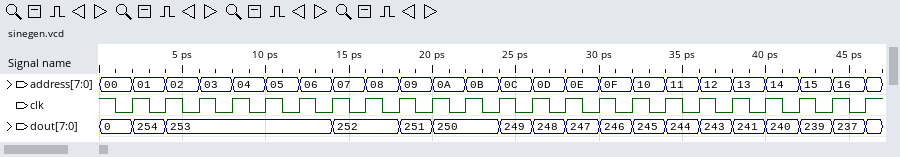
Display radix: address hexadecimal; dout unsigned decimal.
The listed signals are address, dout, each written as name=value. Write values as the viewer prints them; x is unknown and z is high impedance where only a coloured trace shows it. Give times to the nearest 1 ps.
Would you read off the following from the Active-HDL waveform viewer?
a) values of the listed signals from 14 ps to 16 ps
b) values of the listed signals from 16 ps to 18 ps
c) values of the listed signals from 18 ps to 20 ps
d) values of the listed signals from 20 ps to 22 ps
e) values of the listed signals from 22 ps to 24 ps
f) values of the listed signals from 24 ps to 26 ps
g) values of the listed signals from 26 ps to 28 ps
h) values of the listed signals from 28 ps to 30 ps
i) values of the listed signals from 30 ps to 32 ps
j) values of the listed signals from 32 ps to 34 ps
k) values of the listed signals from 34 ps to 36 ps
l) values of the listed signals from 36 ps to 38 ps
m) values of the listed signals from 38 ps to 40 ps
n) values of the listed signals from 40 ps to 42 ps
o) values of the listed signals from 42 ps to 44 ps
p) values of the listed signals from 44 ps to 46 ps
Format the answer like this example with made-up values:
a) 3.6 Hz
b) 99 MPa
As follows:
a) address=07, dout=252
b) address=08, dout=252
c) address=09, dout=251
d) address=0A, dout=250
e) address=0B, dout=250
f) address=0C, dout=249
g) address=0D, dout=248
h) address=0E, dout=247
i) address=0F, dout=246
j) address=10, dout=245
k) address=11, dout=244
l) address=12, dout=243
m) address=13, dout=241
n) address=14, dout=240
o) address=15, dout=239
p) address=16, dout=237
